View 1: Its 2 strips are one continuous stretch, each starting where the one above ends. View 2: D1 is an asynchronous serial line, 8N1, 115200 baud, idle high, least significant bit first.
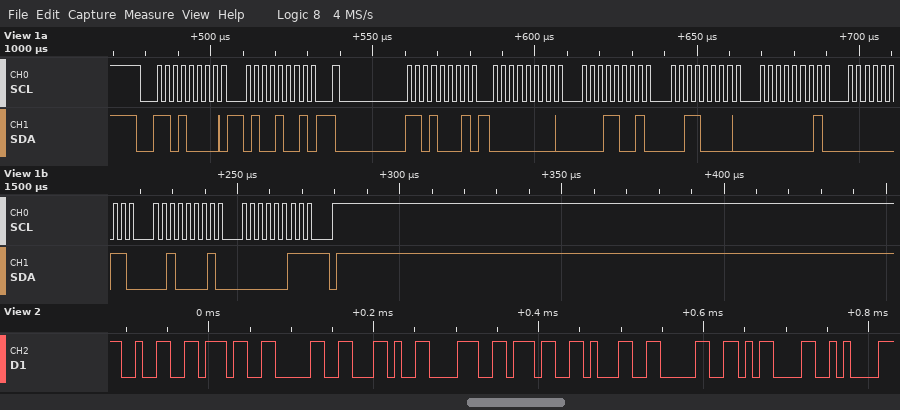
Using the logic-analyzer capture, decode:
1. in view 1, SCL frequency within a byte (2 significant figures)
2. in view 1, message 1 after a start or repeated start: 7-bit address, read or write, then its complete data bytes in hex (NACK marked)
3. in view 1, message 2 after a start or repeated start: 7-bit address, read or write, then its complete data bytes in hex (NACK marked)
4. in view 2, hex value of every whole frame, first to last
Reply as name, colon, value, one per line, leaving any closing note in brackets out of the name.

in view 1, SCL frequency within a byte: 400 kHz
in view 1, message 1 after a start or repeated start: 7-bit address, read or write, then its complete data bytes in hex: 0x68 write: 49
in view 1, message 2 after a start or repeated start: 7-bit address, read or write, then its complete data bytes in hex: 0x68 read: 00 19 30 01 03 21 03 NACK
in view 2, hex value of every whole frame, first to last: 32 37 30 2C 38 37 31 30 0D 0A
